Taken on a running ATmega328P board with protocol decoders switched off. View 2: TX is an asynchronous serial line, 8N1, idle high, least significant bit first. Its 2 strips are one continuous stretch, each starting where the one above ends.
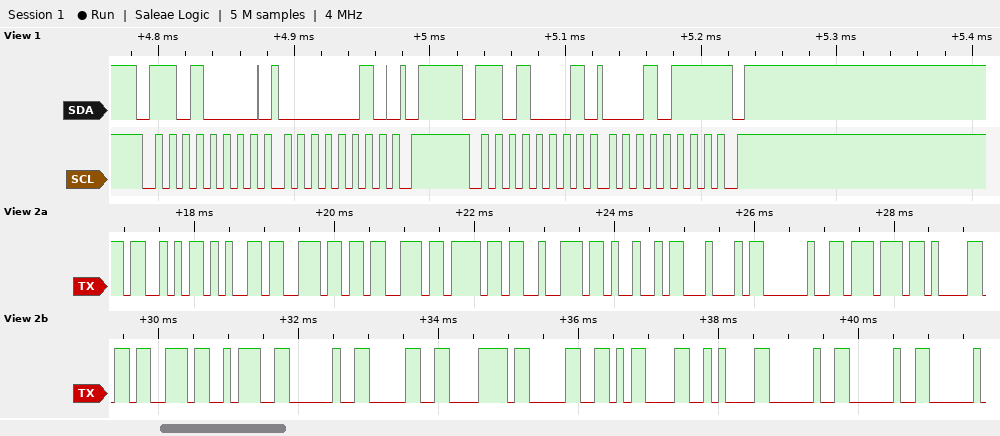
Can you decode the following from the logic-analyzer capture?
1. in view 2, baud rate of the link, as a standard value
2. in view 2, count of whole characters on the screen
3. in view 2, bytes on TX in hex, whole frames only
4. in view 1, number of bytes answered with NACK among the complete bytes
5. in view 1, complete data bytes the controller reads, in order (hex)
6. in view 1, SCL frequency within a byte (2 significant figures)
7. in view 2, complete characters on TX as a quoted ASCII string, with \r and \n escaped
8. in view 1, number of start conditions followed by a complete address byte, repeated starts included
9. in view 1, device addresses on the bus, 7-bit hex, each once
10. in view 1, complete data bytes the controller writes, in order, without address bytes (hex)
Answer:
9600 baud
21
53 65 6E 73 6F 72 49 44 20 77 61 73 3A 20 30 78 30 0D 0A 20 20
1
17
100 kHz
"SensorID was: 0x0\r\n  "
2
0x68
02
